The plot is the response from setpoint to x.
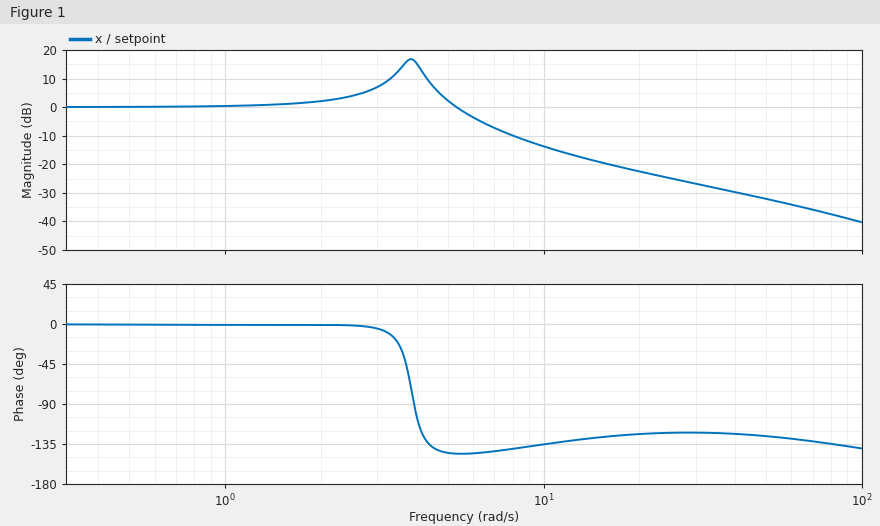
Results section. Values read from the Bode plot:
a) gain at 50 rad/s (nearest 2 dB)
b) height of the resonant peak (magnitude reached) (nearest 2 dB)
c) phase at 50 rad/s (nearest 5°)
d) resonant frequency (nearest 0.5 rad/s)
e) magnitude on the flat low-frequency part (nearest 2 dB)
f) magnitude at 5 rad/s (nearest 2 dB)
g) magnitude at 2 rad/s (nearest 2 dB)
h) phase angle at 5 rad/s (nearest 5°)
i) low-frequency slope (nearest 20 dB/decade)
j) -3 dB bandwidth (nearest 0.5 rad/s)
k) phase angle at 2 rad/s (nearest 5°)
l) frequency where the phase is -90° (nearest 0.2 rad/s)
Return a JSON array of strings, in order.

["-32 dB", "16 dB", "-125°", "4.0 rad/s", "0 dB", "2 dB", "2 dB", "-145°", "0 dB/decade", "6.0 rad/s", "0°", "4.0 rad/s"]
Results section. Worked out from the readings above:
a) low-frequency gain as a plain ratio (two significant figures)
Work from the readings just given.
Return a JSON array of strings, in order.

["1.0"]
